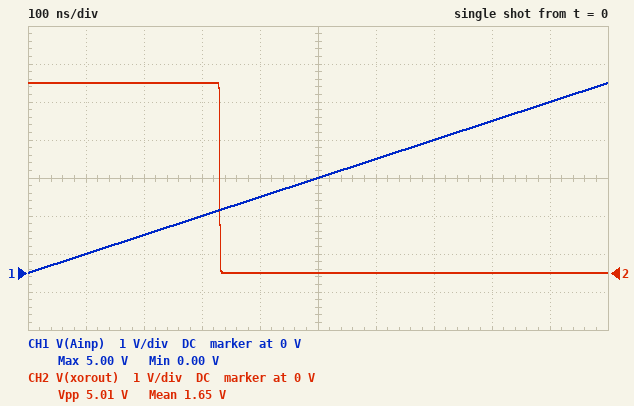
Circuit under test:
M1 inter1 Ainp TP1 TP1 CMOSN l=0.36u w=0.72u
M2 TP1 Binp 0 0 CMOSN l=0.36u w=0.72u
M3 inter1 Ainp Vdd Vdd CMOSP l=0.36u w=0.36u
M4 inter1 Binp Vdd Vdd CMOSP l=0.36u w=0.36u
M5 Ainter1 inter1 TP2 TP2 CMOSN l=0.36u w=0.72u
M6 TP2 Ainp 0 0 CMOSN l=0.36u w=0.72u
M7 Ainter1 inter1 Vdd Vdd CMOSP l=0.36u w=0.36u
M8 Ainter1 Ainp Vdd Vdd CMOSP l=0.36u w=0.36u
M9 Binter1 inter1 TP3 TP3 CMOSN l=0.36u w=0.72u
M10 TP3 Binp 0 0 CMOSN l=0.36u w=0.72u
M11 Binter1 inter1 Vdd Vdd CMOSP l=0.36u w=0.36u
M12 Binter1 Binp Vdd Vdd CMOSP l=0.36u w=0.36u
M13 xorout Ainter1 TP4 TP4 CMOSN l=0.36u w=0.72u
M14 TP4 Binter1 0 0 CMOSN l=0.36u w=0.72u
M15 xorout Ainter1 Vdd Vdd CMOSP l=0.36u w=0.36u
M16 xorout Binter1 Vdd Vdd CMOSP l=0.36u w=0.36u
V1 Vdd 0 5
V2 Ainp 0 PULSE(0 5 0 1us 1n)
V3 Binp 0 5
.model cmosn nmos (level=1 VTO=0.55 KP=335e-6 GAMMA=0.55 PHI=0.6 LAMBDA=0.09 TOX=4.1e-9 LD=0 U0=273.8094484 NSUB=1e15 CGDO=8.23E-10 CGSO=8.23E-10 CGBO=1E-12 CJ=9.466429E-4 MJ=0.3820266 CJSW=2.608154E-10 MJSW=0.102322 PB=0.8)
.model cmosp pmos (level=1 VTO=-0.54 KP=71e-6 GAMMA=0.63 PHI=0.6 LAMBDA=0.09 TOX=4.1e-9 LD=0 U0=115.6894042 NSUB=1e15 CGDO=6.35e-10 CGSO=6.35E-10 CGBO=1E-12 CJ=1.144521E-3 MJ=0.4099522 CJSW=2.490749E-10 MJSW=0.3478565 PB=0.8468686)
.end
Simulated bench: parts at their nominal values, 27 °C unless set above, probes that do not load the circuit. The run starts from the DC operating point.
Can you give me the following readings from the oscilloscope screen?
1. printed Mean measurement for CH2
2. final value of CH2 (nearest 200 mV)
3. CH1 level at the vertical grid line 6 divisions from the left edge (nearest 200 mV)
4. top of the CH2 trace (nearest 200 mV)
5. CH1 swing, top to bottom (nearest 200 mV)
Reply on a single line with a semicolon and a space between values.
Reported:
1.65 V; 0 V; 3.0 V; 5.0 V; 5.0 V
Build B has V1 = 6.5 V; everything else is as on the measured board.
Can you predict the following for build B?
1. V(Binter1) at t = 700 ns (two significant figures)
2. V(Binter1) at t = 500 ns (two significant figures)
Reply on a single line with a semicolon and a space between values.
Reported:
6.5 V; 6.3 V
